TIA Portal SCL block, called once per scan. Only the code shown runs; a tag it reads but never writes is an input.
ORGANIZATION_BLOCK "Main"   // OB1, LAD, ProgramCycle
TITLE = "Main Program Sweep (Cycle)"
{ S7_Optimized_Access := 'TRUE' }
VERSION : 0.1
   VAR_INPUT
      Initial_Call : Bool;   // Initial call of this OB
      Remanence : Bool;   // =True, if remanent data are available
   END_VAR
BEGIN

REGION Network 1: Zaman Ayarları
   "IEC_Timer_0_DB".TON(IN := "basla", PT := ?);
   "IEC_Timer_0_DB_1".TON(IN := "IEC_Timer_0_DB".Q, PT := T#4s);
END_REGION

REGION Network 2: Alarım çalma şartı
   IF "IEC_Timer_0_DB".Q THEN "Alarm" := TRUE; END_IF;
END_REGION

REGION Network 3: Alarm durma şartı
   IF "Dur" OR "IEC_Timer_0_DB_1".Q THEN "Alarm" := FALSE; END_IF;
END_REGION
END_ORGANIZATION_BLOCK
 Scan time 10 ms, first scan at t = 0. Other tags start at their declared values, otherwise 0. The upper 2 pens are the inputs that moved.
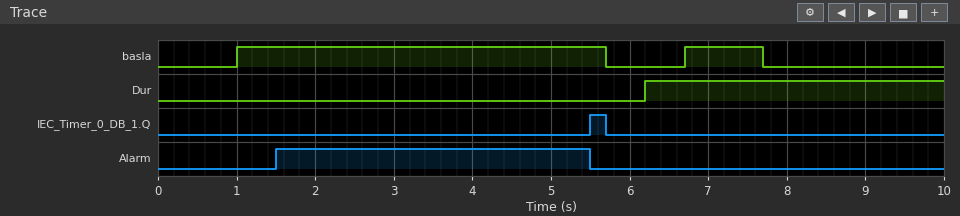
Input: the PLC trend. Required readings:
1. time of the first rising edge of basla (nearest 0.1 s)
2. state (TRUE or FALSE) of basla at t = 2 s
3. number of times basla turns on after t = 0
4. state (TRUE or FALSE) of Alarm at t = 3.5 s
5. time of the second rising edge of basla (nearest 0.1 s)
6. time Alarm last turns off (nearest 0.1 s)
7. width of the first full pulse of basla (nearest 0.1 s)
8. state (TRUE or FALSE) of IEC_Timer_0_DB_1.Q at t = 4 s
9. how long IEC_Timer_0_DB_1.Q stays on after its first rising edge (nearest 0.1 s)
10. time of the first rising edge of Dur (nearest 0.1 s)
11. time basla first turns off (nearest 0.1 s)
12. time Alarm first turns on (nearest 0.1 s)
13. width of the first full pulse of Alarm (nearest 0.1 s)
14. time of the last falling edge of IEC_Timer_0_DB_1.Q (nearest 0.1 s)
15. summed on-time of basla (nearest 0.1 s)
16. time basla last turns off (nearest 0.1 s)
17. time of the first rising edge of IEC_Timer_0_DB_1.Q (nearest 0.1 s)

1.0 s
TRUE
2
TRUE
6.7 s
5.5 s
4.7 s
FALSE
0.2 s
6.2 s
5.7 s
1.5 s
4.0 s
5.7 s
5.7 s
7.7 s
5.5 s
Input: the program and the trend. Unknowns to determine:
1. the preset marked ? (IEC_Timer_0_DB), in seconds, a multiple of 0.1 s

0.5 s
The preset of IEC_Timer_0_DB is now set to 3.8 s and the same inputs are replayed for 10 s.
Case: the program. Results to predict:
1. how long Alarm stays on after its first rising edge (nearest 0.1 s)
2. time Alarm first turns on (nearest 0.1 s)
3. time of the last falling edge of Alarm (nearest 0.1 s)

1.4 s
4.8 s
6.2 s
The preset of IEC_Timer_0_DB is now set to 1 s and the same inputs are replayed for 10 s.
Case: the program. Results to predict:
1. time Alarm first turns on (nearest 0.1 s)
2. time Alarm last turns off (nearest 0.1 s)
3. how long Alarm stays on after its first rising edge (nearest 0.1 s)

2.0 s
6.2 s
4.2 s
